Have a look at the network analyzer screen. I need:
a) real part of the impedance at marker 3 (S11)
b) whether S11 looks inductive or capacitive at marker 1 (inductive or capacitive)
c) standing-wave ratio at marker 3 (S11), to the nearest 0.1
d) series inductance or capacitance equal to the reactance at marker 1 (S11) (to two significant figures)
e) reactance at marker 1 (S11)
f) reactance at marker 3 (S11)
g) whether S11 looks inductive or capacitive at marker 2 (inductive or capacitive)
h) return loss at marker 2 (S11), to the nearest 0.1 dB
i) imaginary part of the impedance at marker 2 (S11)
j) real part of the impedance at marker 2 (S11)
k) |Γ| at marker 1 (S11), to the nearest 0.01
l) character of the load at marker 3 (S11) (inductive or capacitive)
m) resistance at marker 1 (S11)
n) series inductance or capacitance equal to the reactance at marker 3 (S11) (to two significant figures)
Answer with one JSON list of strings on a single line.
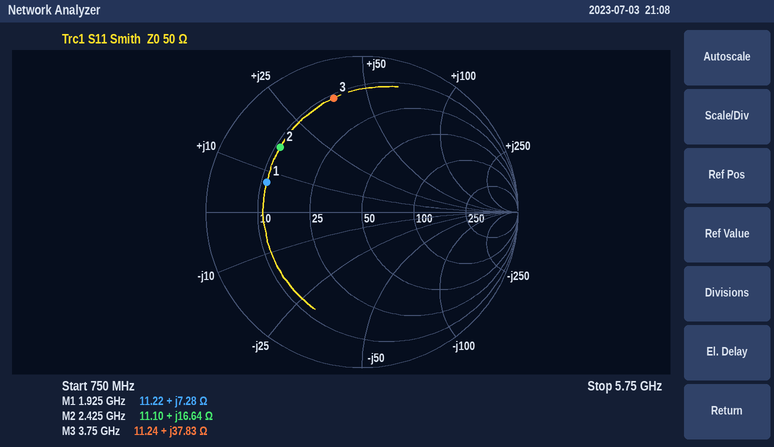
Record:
["11.24 Ω", "inductive", "7.1", "600 pH", "+7.28 Ω", "+37.83 Ω", "inductive", "3.5 dB", "+16.64 Ω", "11.10 Ω", "0.64", "inductive", "11.22 Ω", "1.6 nH"]
